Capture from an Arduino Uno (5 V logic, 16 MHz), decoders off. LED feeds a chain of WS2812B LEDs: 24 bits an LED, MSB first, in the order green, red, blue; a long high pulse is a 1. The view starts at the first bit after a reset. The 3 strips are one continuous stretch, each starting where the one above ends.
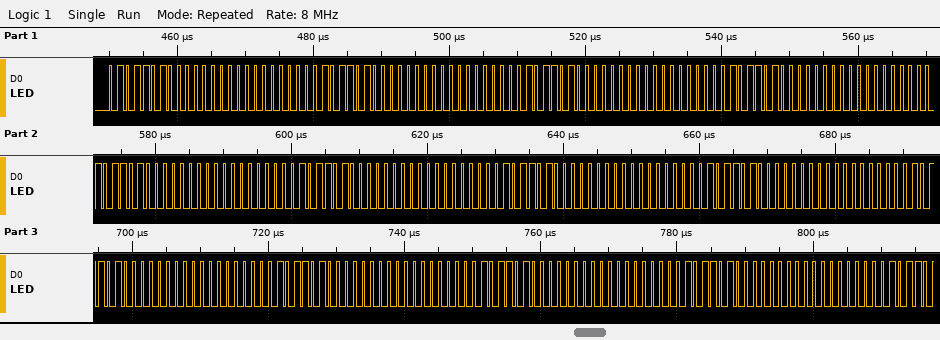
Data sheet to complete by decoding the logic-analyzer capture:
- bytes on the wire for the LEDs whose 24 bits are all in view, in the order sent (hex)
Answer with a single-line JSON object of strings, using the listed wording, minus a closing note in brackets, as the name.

{"bytes on the wire for the LEDs whose 24 bits are all in view, in the order sent": "5A 00 00 5A 00 00 5A 00 00 5A 00 00 5A 00 00 5A 00 00 5A 00 00 5A 00 00 5A 00 00 5A 00 00 5A 00 00 5A 00 00"}
